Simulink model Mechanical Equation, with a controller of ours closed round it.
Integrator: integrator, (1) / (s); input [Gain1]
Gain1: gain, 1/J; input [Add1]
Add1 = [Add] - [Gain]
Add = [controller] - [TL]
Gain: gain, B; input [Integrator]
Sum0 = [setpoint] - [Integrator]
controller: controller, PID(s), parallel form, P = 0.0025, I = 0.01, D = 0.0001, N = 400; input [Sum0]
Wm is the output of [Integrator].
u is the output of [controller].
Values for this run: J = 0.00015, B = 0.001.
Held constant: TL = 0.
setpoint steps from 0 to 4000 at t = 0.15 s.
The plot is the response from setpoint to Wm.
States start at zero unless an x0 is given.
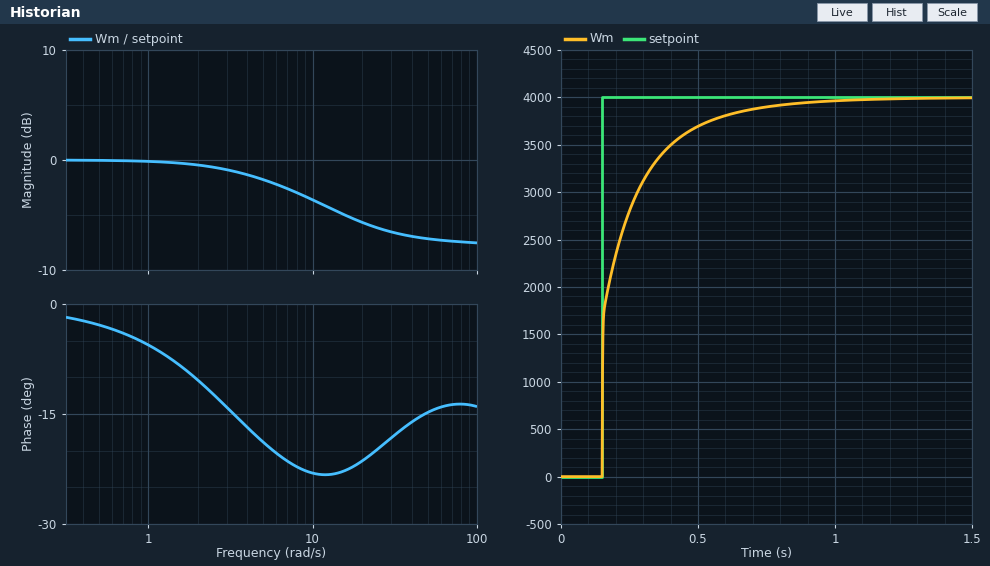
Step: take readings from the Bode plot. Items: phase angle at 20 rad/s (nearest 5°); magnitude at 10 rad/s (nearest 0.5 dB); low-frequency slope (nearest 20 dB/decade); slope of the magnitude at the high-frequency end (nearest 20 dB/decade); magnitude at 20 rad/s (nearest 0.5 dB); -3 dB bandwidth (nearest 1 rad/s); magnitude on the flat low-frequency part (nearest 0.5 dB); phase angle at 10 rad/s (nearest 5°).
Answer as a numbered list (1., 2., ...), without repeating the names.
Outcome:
1. -20°
2. -3.5 dB
3. 0 dB/decade
4. 0 dB/decade
5. -5.5 dB
6. 8 rad/s
7. 0.0 dB
8. -25°
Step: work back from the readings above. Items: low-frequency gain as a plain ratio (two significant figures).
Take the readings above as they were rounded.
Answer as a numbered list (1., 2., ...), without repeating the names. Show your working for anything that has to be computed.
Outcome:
1. 10^(0 / 20) = 1.0
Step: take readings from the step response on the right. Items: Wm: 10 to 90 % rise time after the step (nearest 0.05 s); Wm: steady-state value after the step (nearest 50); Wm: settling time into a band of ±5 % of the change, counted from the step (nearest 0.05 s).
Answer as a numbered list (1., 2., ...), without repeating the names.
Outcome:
1. 0.30 s
2. 4000
3. 0.45 s
